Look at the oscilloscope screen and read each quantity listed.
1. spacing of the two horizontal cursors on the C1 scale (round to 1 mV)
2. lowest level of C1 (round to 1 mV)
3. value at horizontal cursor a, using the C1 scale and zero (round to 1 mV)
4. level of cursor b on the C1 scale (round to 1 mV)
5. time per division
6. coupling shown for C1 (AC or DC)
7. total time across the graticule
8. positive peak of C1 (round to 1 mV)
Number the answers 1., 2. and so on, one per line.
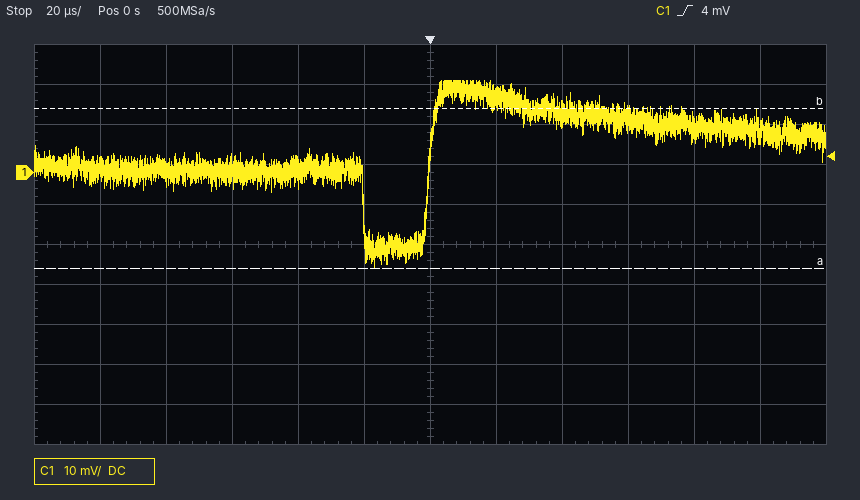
1. 40 mV
2. -24 mV
3. -24 mV
4. 16 mV
5. 20 µs
6. DC
7. 240 µs
8. 23 mV
